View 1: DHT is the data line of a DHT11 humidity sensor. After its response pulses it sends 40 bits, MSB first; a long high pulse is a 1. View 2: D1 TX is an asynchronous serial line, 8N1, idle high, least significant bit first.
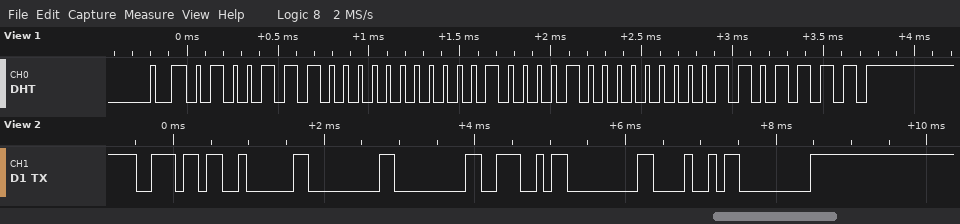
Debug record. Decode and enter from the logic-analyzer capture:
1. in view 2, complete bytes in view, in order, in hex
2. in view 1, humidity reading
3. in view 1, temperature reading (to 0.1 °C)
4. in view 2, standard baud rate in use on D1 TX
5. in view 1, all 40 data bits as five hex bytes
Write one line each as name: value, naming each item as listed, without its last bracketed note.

in view 2, complete bytes in view, in order, in hex: 0x6E 0x02 0x00 0x00 0x4E 0x00 0x48 0x00
in view 1, humidity reading: 78 %
in view 1, temperature reading: 33.0 °C
in view 2, standard baud rate in use on D1 TX: 9600 baud
in view 1, all 40 data bits as five hex bytes: 4E 00 21 00 6F
